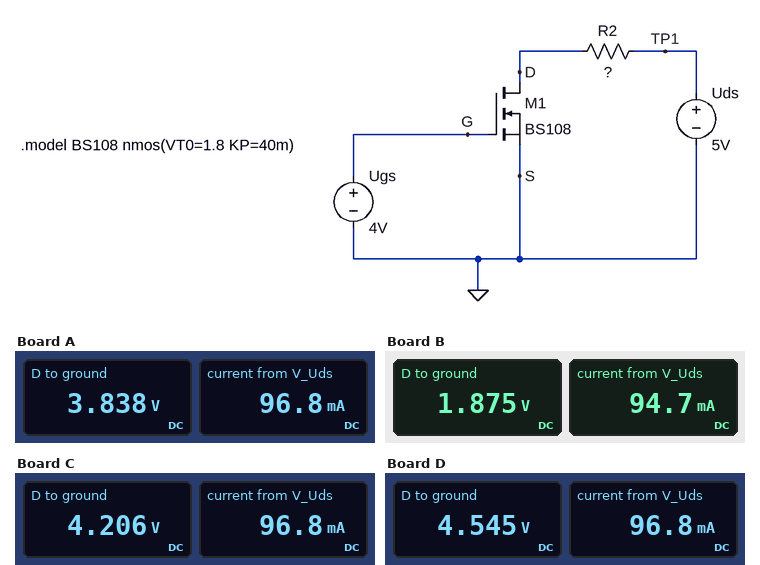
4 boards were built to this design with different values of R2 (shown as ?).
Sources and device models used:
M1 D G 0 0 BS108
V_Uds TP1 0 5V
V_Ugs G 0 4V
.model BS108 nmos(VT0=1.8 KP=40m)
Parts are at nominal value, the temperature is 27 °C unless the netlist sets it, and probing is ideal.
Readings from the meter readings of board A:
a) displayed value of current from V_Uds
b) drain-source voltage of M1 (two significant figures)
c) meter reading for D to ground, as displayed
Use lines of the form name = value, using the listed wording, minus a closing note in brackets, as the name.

displayed value of current from V_Uds = 96.8 mA
drain-source voltage of M1 = 3.8 V
meter reading for D to ground, as displayed = 3.838 V
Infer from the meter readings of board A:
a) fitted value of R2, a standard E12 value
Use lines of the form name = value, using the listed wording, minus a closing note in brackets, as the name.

fitted value of R2, a standard E12 value = 12 Ω
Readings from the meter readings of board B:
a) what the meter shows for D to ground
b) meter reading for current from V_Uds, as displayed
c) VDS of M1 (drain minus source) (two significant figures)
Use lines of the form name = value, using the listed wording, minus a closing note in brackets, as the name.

what the meter shows for D to ground = 1.875 V
meter reading for current from V_Uds, as displayed = 94.7 mA
VDS of M1 (drain minus source) = 1.9 V
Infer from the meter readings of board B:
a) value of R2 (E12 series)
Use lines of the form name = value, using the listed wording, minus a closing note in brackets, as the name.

value of R2 = 33 Ω
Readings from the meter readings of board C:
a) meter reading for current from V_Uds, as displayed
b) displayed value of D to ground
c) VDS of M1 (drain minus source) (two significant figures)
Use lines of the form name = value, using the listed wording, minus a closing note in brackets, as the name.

meter reading for current from V_Uds, as displayed = 96.8 mA
displayed value of D to ground = 4.206 V
VDS of M1 (drain minus source) = 4.2 V
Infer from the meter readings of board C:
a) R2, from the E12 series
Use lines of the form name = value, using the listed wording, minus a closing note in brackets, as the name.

R2, from the E12 series = 8.2 Ω
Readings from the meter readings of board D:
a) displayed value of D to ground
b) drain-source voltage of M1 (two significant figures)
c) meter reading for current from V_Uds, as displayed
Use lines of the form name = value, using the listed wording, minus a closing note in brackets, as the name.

displayed value of D to ground = 4.545 V
drain-source voltage of M1 = 4.5 V
meter reading for current from V_Uds, as displayed = 96.8 mA
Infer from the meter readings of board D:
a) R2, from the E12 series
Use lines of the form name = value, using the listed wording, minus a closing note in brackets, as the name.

R2, from the E12 series = 4.7 Ω
